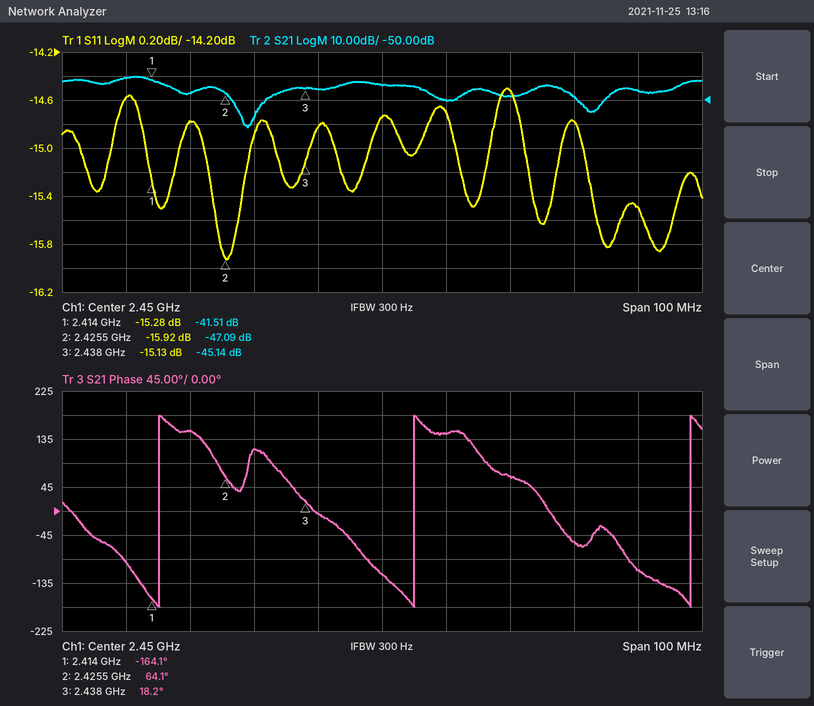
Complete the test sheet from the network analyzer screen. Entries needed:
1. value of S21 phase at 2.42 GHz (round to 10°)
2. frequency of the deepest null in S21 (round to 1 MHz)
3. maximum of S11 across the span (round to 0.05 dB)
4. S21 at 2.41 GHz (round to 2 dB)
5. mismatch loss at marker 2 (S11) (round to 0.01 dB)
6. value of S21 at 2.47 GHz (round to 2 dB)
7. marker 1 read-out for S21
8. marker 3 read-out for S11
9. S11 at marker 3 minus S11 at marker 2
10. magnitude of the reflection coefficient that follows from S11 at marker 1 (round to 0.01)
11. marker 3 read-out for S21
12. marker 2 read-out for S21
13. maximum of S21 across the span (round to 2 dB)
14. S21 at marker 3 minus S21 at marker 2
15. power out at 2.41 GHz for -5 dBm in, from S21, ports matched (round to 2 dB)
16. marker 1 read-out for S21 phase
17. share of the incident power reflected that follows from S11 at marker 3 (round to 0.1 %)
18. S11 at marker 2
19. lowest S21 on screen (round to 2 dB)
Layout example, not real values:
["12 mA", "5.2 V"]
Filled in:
["150°", "2.429 GHz", "-14.50 dB", "-40 dB", "0.11 dB", "-48 dB", "-41.51 dB", "-15.13 dB", "0.79 dB", "0.17", "-45.14 dB", "-47.09 dB", "-40 dB", "1.95 dB", "-46 dBm", "-164.1°", "3.1 %", "-15.92 dB", "-62 dB"]
